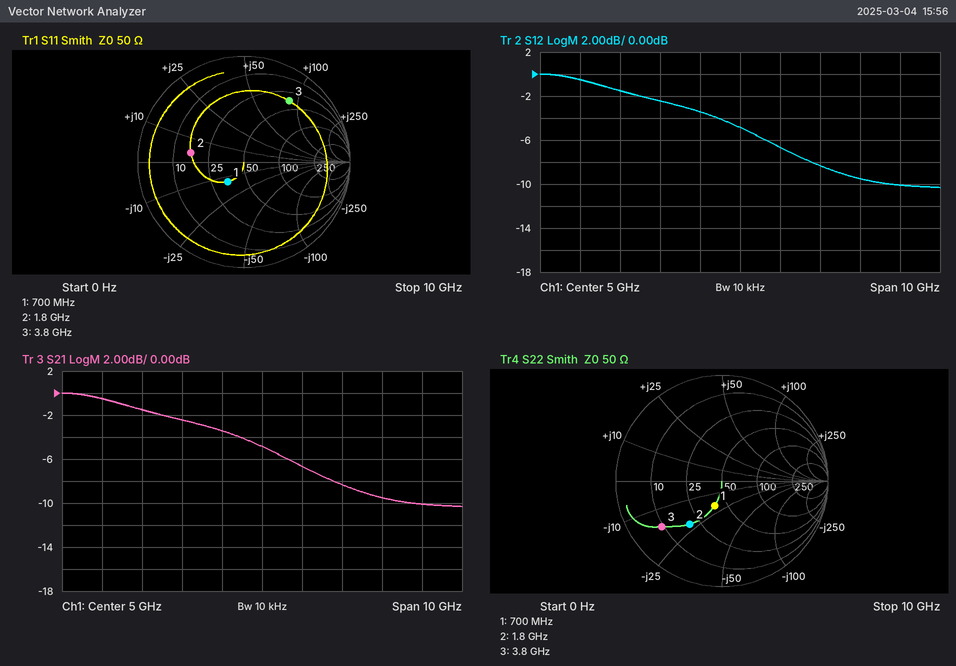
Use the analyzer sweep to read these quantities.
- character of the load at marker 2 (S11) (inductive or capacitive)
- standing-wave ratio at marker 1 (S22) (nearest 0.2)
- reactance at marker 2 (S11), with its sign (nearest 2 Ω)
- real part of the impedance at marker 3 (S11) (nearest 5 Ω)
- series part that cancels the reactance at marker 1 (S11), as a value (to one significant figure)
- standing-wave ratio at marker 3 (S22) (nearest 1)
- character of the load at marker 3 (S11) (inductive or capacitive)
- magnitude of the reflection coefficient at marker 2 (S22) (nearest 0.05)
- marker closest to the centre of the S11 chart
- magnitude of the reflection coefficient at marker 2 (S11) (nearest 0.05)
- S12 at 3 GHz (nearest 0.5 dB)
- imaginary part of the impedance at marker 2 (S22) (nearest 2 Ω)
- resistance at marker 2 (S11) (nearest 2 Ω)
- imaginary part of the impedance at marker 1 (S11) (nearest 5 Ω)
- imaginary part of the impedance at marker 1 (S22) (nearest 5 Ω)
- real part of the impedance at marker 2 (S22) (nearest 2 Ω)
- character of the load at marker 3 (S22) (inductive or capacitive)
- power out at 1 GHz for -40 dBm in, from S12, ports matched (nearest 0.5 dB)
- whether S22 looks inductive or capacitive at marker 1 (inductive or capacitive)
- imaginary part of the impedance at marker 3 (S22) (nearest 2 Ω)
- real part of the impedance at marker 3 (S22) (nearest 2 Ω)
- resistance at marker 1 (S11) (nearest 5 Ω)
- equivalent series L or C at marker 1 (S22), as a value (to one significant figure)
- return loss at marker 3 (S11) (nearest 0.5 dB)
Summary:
inductive
1.6
+4 Ω
35 Ω
3 nH
6
inductive
0.50
marker 1
0.50
-2.5 dB
-22 Ω
16 Ω
-15 Ω
-20 Ω
20 Ω
capacitive
-40.5 dBm
capacitive
-16 Ω
10 Ω
35 Ω
10 pF
3.0 dB
